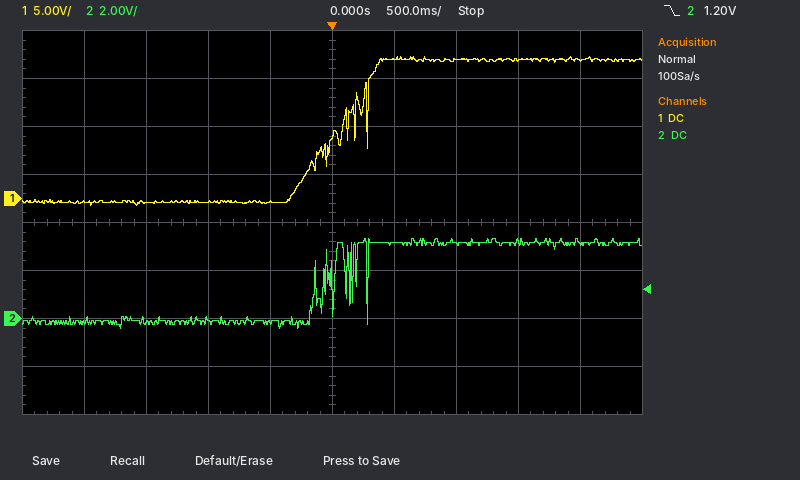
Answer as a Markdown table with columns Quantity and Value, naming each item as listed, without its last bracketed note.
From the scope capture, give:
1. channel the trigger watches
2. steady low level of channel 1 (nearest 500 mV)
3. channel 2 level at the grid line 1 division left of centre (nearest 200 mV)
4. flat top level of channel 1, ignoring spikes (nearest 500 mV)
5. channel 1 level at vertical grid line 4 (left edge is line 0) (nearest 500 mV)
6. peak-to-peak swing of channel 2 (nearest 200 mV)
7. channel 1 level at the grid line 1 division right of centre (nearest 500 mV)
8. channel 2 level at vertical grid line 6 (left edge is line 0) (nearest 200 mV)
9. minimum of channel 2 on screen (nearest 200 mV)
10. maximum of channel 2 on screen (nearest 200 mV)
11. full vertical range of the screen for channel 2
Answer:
| Quantity | Value |
|---|---|
| channel the trigger watches | channel 2 |
| steady low level of channel 1 | -500 mV |
| channel 2 level at the grid line 1 division left of centre | -200 mV |
| flat top level of channel 1, ignoring spikes | 14.5 V |
| channel 1 level at vertical grid line 4 (left edge is line 0) | -500 mV |
| peak-to-peak swing of channel 2 | 3.8 V |
| channel 1 level at the grid line 1 division right of centre | 14.5 V |
| channel 2 level at vertical grid line 6 (left edge is line 0) | 3.2 V |
| minimum of channel 2 on screen | -400 mV |
| maximum of channel 2 on screen | 3.4 V |
| full vertical range of the screen for channel 2 | 16 V |
